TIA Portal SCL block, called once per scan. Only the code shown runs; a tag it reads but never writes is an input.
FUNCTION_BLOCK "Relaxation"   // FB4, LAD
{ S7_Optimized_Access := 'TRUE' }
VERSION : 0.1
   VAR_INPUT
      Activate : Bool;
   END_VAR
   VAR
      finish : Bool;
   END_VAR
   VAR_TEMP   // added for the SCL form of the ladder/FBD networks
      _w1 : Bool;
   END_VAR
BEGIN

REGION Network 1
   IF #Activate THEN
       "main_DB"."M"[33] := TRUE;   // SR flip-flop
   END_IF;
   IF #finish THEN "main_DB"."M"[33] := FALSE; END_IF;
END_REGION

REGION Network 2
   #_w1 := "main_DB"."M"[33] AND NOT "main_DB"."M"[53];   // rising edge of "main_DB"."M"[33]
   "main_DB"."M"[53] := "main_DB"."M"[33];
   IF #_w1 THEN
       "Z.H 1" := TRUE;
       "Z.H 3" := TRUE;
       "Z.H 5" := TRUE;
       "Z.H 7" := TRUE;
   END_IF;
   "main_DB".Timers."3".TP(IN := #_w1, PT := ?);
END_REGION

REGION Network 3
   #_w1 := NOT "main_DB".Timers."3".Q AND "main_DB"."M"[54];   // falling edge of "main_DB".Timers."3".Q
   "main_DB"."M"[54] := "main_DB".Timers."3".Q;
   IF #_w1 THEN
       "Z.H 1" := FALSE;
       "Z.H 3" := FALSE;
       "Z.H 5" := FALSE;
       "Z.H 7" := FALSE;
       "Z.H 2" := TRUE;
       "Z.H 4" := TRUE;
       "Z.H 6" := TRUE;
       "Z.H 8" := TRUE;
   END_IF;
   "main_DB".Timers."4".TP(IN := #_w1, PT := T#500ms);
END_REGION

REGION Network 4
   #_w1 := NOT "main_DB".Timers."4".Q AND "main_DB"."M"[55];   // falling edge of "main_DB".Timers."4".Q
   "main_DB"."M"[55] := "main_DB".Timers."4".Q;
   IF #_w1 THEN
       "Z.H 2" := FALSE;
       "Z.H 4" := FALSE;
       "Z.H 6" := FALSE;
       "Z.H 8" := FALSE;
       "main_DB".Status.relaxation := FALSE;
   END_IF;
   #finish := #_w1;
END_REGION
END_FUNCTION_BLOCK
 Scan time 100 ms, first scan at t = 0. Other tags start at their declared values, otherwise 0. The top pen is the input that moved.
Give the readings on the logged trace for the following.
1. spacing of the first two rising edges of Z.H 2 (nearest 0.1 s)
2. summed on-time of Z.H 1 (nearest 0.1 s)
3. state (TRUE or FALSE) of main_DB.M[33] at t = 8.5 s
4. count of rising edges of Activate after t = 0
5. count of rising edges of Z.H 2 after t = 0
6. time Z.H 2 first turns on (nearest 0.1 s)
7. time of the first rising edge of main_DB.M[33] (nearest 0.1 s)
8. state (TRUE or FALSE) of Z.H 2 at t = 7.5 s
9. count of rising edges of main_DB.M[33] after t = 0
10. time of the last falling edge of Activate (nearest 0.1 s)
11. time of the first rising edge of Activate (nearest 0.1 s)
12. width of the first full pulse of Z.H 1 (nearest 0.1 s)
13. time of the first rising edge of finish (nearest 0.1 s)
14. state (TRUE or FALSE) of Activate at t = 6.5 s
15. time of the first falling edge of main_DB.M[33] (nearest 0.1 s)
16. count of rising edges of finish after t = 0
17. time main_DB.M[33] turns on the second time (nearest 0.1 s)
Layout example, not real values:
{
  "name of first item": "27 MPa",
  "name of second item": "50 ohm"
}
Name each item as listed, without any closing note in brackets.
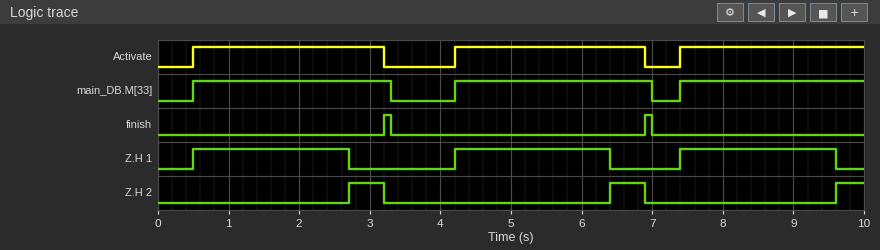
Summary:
{
  "spacing of the first two rising edges of Z.H 2": "3.7 s",
  "summed on-time of Z.H 1": "6.6 s",
  "state (TRUE or FALSE) of main_DB.M[33] at t = 8.5 s": "TRUE",
  "count of rising edges of Activate after t = 0": "3",
  "count of rising edges of Z.H 2 after t = 0": "3",
  "time Z.H 2 first turns on": "2.7 s",
  "time of the first rising edge of main_DB.M[33]": "0.5 s",
  "state (TRUE or FALSE) of Z.H 2 at t = 7.5 s": "FALSE",
  "count of rising edges of main_DB.M[33] after t = 0": "3",
  "time of the last falling edge of Activate": "6.9 s",
  "time of the first rising edge of Activate": "0.5 s",
  "width of the first full pulse of Z.H 1": "2.2 s",
  "time of the first rising edge of finish": "3.2 s",
  "state (TRUE or FALSE) of Activate at t = 6.5 s": "TRUE",
  "time of the first falling edge of main_DB.M[33]": "3.3 s",
  "count of rising edges of finish after t = 0": "2",
  "time main_DB.M[33] turns on the second time": "4.2 s"
}
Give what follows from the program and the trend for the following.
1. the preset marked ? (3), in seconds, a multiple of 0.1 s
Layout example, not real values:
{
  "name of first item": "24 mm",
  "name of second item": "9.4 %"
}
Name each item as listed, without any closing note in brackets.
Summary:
{
  "the preset marked ? (3), in seconds, a multiple of 0.1 s": "2.2 s"
}
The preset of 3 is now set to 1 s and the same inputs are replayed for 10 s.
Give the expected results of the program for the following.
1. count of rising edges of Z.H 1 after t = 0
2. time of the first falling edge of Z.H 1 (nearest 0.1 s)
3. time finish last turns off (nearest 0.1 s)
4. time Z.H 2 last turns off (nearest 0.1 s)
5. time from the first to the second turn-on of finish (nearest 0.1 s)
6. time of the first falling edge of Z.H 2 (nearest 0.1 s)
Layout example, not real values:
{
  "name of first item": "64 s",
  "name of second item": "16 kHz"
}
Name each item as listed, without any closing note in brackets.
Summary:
{
  "count of rising edges of Z.H 1 after t = 0": "6",
  "time of the first falling edge of Z.H 1": "1.5 s",
  "time finish last turns off": "9.2 s",
  "time Z.H 2 last turns off": "9.1 s",
  "time from the first to the second turn-on of finish": "1.7 s",
  "time of the first falling edge of Z.H 2": "2.0 s"
}
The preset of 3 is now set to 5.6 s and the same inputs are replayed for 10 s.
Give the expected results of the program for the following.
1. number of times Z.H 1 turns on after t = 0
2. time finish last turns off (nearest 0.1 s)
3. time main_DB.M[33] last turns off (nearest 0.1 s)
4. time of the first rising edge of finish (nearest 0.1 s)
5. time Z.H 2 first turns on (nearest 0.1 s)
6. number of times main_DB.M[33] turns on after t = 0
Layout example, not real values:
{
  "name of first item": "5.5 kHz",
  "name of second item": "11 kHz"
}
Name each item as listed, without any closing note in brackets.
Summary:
{
  "number of times Z.H 1 turns on after t = 0": "2",
  "time finish last turns off": "6.7 s",
  "time main_DB.M[33] last turns off": "6.7 s",
  "time of the first rising edge of finish": "6.6 s",
  "time Z.H 2 first turns on": "6.1 s",
  "number of times main_DB.M[33] turns on after t = 0": "2"
}
